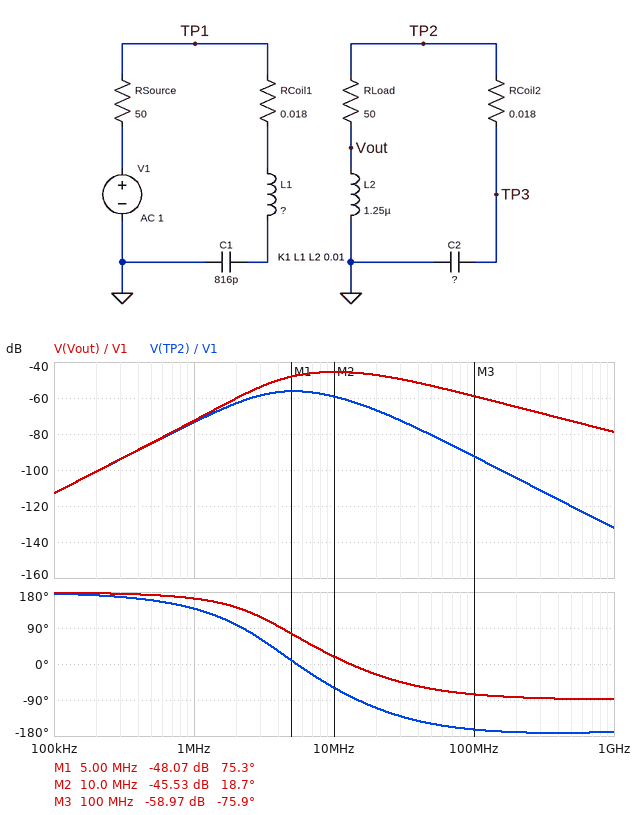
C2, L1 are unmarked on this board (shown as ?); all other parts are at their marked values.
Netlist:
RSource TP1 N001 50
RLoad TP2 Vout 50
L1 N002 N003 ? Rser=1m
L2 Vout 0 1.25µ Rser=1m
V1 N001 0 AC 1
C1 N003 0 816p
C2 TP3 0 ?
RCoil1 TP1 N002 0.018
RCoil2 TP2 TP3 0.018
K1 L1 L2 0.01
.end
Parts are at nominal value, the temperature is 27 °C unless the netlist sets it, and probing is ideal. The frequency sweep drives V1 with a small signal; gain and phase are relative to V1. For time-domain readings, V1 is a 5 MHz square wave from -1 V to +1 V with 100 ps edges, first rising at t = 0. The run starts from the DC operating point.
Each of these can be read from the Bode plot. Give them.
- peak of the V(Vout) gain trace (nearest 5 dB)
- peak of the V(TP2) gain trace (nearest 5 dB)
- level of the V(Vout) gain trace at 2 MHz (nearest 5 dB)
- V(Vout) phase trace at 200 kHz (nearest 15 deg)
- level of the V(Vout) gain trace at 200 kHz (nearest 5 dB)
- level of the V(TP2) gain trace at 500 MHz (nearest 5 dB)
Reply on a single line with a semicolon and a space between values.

-45 dB; -55 dB; -60 dB; 180 deg; -100 dB; -120 dB
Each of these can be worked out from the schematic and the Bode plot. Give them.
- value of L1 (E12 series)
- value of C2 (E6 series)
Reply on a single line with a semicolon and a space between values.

390 nH; 1.5 nF
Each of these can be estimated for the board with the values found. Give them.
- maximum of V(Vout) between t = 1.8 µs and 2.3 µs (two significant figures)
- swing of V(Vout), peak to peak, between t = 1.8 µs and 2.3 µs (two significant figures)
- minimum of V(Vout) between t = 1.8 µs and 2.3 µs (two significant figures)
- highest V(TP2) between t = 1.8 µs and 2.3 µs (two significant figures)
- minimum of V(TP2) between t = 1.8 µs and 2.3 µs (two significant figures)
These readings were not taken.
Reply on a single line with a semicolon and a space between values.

8.2 mV; 16 mV; -8.2 mV; 2.1 mV; -2.1 mV
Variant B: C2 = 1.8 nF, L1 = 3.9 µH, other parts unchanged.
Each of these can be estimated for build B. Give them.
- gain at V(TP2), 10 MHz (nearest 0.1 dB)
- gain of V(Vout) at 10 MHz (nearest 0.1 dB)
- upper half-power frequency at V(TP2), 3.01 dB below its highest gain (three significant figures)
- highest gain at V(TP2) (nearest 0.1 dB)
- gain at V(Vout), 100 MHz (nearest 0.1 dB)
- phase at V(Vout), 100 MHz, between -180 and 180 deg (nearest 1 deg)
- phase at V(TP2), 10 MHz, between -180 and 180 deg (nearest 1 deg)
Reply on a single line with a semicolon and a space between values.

-64.2 dB; -49.0 dB; 4.01 MHz; -46.3 dB; -68.9 dB; -86 deg; -132 deg
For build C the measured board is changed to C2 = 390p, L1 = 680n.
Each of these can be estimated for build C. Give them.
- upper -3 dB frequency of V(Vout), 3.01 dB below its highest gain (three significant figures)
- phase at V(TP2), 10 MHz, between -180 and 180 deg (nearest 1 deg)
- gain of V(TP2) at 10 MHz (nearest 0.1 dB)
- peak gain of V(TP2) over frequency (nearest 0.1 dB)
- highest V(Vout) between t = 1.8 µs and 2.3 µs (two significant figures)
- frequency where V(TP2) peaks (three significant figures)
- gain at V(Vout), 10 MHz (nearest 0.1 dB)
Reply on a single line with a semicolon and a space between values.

11.8 MHz; -62 deg; -43.3 dB; -40.5 dB; 12 mV; 7.11 MHz; -39.3 dB
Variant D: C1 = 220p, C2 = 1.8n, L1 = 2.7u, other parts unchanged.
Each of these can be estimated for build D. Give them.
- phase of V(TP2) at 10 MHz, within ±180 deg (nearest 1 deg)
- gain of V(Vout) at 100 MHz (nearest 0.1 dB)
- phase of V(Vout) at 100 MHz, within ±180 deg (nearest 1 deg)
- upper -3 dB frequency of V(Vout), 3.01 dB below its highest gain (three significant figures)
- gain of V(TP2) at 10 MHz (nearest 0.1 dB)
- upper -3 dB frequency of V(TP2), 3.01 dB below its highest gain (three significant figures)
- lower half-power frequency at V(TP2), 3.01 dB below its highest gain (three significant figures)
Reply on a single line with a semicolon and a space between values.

-117 deg; -67.2 dB; -86 deg; 8.39 MHz; -59.3 dB; 7.73 MHz; 4.91 MHz
